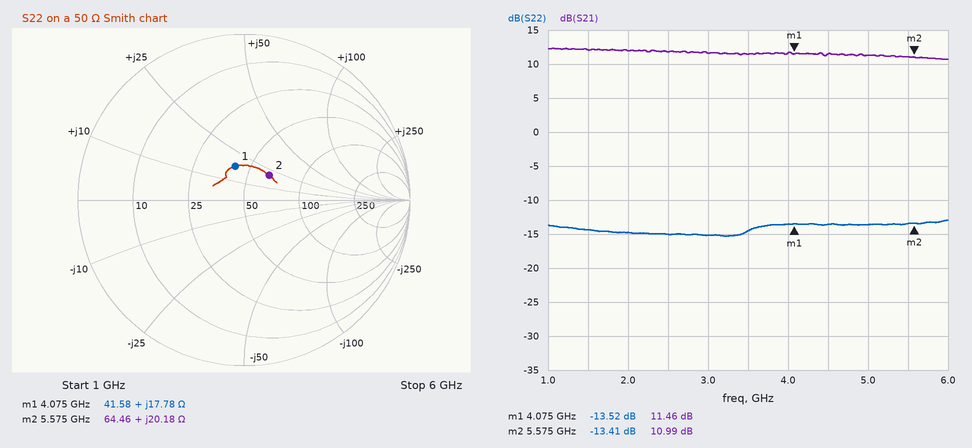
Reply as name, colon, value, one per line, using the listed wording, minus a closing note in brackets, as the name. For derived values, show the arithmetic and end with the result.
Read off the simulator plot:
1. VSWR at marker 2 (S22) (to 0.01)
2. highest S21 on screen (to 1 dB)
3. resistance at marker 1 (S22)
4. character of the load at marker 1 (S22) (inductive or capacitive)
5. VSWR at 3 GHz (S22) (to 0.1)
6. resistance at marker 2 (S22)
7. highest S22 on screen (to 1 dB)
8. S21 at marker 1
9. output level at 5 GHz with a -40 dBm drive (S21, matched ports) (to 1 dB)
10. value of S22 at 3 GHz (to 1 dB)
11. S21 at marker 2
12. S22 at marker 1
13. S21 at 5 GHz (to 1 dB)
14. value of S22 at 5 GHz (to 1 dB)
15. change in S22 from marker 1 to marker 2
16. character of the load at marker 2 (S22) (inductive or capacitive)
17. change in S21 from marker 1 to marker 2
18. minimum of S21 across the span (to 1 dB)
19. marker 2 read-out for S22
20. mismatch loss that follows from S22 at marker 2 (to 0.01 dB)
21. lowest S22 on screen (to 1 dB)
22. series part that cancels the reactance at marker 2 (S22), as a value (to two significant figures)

VSWR at marker 2 (S22): 1.54
highest S21 on screen: 12 dB
resistance at marker 1: 41.58 Ω
character of the load at marker 1 (S22): inductive
VSWR at 3 GHz (S22): |Γ| = 10^(-15/20) = 0.1778; VSWR = (1 + 0.1778)/(1 − 0.1778) ≈ 1.4
resistance at marker 2: 64.46 Ω
highest S22 on screen: -13 dB
S21 at marker 1: 11.46 dB
output level at 5 GHz with a -40 dBm drive (S21, matched ports): -40 dBm + (11 dB) = -29 dBm
value of S22 at 3 GHz: -15 dB
S21 at marker 2: 10.99 dB
S22 at marker 1: -13.52 dB
S21 at 5 GHz: 11 dB
value of S22 at 5 GHz: -14 dB
change in S22 from marker 1 to marker 2: -13.41 − (-13.52) = 0.11 dB
character of the load at marker 2 (S22): inductive
change in S21 from marker 1 to marker 2: 10.99 − (11.46) = -0.47 dB
minimum of S21 across the span: 11 dB
marker 2 read-out for S22: -13.41 dB
mismatch loss that follows from S22 at marker 2: −10 log10(1 − 10^(-13.41/10)) ≈ 0.20 dB
lowest S22 on screen: -15 dB
series part that cancels the reactance at marker 2 (S22), as a value: C = 1/(2π × 5.575 GHz × 20.18 Ω) ≈ 1.4 pF
